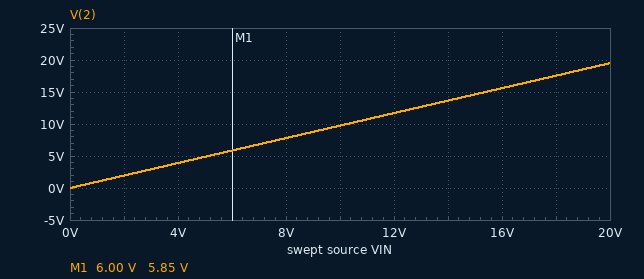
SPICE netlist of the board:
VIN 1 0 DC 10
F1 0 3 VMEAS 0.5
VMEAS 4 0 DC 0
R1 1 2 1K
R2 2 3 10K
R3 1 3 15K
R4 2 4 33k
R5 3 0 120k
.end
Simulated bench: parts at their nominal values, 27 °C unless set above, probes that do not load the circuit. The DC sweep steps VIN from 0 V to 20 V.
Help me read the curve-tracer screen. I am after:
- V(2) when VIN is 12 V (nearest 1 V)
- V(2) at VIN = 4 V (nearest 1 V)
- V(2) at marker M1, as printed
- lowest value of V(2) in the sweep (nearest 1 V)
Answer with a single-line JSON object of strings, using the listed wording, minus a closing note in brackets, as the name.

{"V(2) when VIN is 12 V": "12 V", "V(2) at VIN = 4 V": "4 V", "V(2) at marker M1, as printed": "5.85 V", "lowest value of V(2) in the sweep": "0 V"}
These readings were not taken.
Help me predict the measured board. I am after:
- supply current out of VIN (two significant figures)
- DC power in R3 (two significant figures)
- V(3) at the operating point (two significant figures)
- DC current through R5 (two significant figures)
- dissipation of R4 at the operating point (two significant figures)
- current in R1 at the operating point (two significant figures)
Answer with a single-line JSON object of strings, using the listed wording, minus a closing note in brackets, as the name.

{"supply current out of VIN": "230 µA", "DC power in R3": "3.4 µW", "V(3) at the operating point": "10 V", "DC current through R5": "85 µA", "dissipation of R4 at the operating point": "2.9 mW", "current in R1 at the operating point": "250 µA"}
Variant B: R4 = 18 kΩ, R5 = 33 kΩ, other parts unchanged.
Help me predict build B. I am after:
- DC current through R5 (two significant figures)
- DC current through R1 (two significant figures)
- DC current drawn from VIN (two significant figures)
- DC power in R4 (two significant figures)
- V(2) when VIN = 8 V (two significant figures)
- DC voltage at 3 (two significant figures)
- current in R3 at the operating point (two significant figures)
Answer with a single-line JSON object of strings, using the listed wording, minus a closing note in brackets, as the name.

{"DC current through R5": "290 µA", "DC current through R1": "520 µA", "DC current drawn from VIN": "550 µA", "DC power in R4": "5.0 mW", "V(2) when VIN = 8 V": "7.6 V", "DC voltage at 3": "9.5 V", "current in R3 at the operating point": "31 µA"}
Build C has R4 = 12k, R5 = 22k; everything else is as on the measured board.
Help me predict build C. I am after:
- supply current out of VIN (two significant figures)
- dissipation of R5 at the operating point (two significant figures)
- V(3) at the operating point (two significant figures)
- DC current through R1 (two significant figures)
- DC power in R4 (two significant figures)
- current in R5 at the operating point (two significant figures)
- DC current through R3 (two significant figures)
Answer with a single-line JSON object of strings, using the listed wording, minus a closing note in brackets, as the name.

{"supply current out of VIN": "810 µA", "dissipation of R5 at the operating point": "3.9 mW", "V(3) at the operating point": "9.3 V", "DC current through R1": "760 µA", "DC power in R4": "7.1 mW", "current in R5 at the operating point": "420 µA", "DC current through R3": "46 µA"}
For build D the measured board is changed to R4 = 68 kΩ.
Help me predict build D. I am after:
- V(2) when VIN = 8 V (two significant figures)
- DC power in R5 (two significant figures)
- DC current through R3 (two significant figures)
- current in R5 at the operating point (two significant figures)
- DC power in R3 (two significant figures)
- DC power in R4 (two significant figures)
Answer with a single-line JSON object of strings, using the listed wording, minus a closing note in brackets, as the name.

{"V(2) when VIN = 8 V": "7.9 V", "DC power in R5": "810 µW", "DC current through R3": "9.7 µA", "current in R5 at the operating point": "82 µA", "DC power in R3": "1.4 µW", "DC power in R4": "1.4 mW"}
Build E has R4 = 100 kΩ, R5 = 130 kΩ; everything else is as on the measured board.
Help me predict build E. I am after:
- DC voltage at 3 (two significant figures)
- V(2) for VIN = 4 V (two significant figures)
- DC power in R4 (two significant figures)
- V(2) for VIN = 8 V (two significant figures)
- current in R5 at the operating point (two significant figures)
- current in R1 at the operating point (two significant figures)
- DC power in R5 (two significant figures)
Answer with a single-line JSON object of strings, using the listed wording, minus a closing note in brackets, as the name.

{"DC voltage at 3": "9.8 V", "V(2) for VIN = 4 V": "4.0 V", "DC power in R4": "980 µW", "V(2) for VIN = 8 V": "7.9 V", "current in R5 at the operating point": "75 µA", "current in R1 at the operating point": "110 µA", "DC power in R5": "740 µW"}
